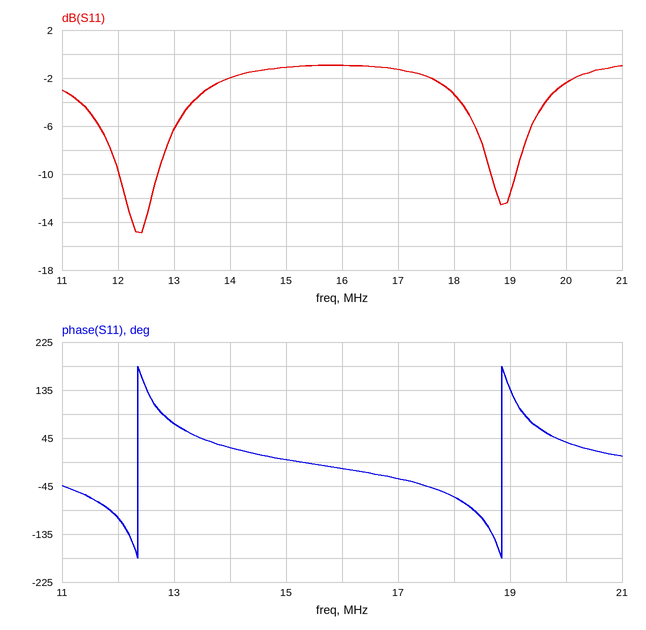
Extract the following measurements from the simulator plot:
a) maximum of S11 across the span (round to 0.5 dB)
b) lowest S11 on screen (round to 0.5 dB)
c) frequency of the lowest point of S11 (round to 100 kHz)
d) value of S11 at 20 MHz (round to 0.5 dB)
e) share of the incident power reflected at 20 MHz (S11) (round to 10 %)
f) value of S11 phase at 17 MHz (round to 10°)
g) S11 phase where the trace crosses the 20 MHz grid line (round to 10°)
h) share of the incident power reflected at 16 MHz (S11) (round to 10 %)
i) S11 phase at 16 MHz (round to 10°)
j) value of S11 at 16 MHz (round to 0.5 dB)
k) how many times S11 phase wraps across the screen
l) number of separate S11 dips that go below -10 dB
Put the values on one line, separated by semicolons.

-1.0 dB; -15.0 dB; 12.4 MHz; -2.5 dB; 60 %; -30°; 40°; 80 %; -10°; -1.0 dB; 2; 2
